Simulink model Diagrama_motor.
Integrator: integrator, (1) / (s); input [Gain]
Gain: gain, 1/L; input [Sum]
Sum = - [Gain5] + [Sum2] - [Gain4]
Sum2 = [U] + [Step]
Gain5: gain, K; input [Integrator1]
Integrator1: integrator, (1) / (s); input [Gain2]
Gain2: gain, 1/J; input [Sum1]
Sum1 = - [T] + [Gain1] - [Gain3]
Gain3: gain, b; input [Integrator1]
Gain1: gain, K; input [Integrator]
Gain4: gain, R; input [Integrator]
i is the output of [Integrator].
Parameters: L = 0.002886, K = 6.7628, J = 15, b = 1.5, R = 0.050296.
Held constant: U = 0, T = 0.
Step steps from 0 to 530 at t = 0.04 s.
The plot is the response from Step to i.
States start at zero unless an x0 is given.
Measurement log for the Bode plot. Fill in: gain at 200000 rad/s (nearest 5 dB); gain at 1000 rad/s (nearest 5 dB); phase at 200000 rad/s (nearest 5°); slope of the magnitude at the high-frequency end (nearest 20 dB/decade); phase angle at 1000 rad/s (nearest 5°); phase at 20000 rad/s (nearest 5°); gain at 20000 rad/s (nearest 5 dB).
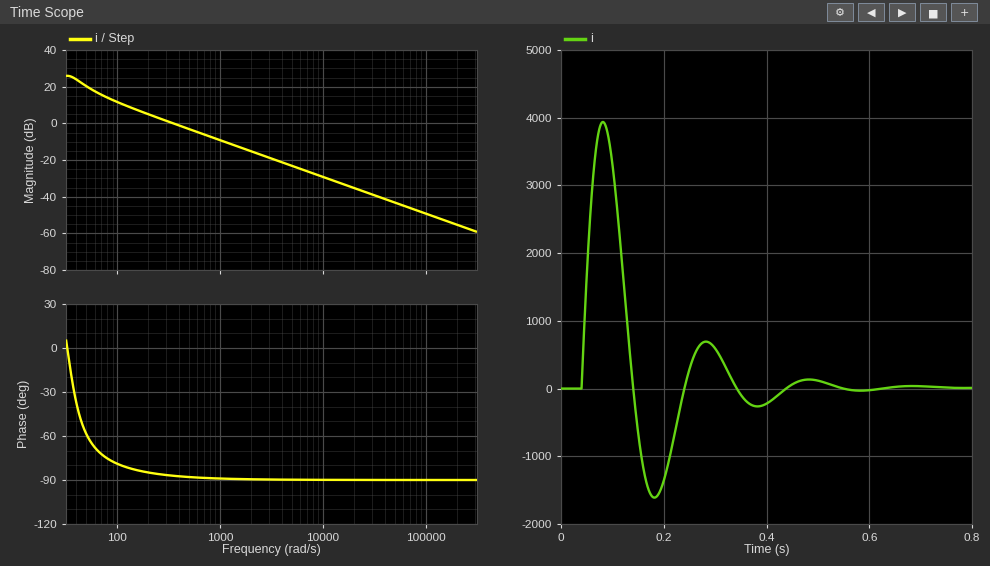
-55 dB
-10 dB
-90°
-20 dB/decade
-90°
-90°
-35 dB
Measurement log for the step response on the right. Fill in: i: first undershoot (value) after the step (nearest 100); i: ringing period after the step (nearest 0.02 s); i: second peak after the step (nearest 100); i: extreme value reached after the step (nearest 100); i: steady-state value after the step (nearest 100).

-1600
0.20 s
700
3900
0
